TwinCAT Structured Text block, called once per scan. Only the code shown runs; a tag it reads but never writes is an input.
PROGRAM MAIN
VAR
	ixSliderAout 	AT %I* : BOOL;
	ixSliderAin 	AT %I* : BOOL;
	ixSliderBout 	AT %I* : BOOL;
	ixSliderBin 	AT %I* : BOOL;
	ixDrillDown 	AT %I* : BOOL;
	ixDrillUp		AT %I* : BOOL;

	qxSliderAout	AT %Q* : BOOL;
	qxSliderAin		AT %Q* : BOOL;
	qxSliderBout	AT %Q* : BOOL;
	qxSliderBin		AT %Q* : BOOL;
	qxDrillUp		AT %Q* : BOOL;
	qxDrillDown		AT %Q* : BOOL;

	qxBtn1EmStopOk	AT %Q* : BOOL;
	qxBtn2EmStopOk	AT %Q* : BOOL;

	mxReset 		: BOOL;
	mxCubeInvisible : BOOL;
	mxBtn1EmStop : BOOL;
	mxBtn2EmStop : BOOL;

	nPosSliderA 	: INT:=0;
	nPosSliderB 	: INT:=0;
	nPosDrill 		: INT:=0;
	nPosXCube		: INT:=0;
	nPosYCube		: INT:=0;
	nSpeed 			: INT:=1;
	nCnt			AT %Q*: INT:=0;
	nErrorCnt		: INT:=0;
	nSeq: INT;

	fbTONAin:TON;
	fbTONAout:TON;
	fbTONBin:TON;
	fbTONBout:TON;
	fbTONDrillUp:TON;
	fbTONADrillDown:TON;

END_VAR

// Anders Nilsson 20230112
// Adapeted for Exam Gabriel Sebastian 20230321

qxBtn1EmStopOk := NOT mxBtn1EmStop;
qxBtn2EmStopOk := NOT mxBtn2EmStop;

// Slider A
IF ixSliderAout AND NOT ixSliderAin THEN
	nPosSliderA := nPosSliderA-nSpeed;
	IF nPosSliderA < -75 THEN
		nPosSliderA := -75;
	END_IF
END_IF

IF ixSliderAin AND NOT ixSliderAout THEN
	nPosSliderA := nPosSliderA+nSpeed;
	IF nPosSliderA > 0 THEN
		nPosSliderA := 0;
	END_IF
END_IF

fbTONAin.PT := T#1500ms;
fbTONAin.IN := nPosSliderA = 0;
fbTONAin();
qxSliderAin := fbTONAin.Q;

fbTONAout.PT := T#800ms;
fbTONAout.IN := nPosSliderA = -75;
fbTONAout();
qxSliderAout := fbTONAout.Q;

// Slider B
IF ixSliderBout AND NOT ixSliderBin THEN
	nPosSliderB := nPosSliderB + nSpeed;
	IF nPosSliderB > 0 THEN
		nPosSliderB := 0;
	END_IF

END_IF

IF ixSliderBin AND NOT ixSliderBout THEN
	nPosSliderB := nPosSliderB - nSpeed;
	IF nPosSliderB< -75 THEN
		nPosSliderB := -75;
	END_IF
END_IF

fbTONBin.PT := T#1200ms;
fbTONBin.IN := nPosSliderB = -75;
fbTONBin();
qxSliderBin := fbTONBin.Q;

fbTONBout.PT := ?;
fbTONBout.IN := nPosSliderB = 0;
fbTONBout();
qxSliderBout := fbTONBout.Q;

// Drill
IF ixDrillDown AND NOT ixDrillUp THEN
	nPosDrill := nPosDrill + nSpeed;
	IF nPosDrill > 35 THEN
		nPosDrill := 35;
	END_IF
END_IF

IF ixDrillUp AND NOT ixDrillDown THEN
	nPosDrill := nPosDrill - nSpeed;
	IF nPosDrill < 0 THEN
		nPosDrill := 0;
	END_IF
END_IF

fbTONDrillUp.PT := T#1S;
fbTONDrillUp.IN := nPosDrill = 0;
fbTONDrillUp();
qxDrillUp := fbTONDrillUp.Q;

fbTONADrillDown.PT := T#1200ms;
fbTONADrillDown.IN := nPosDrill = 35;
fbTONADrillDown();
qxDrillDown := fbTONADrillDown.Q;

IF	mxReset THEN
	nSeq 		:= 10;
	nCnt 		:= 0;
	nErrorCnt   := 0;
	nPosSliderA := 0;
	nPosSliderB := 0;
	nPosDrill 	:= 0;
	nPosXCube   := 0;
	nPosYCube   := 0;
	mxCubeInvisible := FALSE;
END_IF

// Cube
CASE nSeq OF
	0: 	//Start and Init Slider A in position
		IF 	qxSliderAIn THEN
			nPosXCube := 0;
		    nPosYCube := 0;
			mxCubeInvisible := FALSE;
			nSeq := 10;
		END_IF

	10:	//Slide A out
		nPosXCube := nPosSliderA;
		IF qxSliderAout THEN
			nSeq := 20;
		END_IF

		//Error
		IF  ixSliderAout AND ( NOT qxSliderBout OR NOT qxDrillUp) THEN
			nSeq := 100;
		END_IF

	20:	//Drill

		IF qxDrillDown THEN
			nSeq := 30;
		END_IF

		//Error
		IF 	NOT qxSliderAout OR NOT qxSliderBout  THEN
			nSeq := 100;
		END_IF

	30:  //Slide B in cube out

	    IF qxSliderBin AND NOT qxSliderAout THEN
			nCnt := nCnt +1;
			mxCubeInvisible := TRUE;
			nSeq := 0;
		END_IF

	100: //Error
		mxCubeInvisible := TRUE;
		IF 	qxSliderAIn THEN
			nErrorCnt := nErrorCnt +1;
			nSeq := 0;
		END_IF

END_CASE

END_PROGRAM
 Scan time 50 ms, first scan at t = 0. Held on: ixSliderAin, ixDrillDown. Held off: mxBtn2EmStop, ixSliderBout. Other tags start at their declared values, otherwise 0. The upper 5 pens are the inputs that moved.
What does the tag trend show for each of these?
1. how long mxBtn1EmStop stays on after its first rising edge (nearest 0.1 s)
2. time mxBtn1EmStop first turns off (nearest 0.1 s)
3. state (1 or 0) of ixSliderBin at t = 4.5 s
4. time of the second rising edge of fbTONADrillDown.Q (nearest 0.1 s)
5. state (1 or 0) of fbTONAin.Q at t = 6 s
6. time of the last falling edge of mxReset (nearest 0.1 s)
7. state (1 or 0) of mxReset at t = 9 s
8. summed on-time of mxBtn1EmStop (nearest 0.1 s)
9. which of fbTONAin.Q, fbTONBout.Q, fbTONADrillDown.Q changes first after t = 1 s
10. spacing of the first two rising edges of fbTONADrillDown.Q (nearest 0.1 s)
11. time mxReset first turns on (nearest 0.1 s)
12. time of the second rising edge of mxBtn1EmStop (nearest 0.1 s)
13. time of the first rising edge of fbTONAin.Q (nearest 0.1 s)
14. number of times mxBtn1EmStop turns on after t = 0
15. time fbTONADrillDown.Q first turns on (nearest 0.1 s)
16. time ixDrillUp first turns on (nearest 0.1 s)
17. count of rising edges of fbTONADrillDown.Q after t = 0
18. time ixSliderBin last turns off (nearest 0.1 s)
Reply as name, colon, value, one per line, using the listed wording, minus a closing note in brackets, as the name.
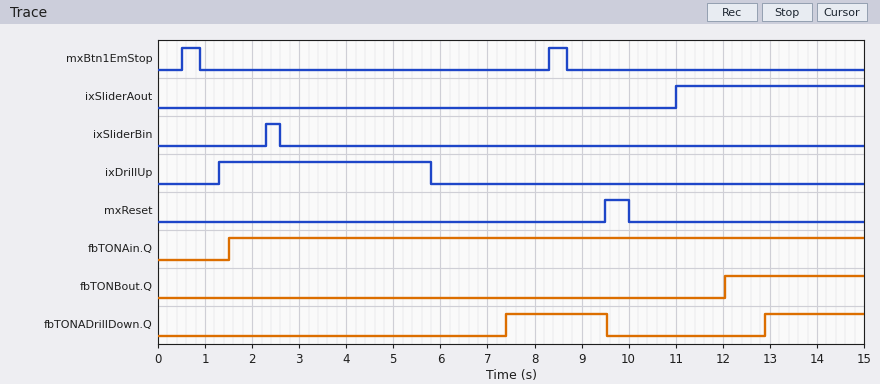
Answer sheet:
how long mxBtn1EmStop stays on after its first rising edge: 0.4 s
time mxBtn1EmStop first turns off: 0.9 s
state (1 or 0) of ixSliderBin at t = 4.5 s: 0
time of the second rising edge of fbTONADrillDown.Q: 12.9 s
state (1 or 0) of fbTONAin.Q at t = 6 s: 1
time of the last falling edge of mxReset: 10.0 s
state (1 or 0) of mxReset at t = 9 s: 0
summed on-time of mxBtn1EmStop: 0.8 s
which of fbTONAin.Q, fbTONBout.Q, fbTONADrillDown.Q changes first after t = 1 s: fbTONAin.Q
spacing of the first two rising edges of fbTONADrillDown.Q: 5.5 s
time mxReset first turns on: 9.5 s
time of the second rising edge of mxBtn1EmStop: 8.3 s
time of the first rising edge of fbTONAin.Q: 1.5 s
number of times mxBtn1EmStop turns on after t = 0: 2
time fbTONADrillDown.Q first turns on: 7.4 s
time ixDrillUp first turns on: 1.3 s
count of rising edges of fbTONADrillDown.Q after t = 0: 2
time ixSliderBin last turns off: 2.6 s
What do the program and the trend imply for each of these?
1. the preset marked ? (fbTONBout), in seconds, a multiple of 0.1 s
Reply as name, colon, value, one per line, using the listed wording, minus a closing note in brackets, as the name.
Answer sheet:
the preset marked ? (fbTONBout), in seconds, a multiple of 0.1 s: 2.5 s
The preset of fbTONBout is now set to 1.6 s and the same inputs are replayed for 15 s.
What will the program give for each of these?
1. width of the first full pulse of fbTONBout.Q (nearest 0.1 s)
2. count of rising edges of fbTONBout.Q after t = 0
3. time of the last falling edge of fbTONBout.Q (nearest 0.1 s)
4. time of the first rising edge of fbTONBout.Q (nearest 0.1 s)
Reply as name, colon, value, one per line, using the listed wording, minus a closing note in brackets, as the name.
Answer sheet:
width of the first full pulse of fbTONBout.Q: 0.7 s
count of rising edges of fbTONBout.Q after t = 0: 2
time of the last falling edge of fbTONBout.Q: 2.3 s
time of the first rising edge of fbTONBout.Q: 1.6 s
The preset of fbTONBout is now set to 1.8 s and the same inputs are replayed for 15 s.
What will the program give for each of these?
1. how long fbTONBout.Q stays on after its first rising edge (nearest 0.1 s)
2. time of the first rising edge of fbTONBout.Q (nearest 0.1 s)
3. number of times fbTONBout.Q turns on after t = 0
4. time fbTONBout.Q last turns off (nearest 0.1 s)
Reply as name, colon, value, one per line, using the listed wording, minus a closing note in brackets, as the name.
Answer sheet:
how long fbTONBout.Q stays on after its first rising edge: 0.5 s
time of the first rising edge of fbTONBout.Q: 1.8 s
number of times fbTONBout.Q turns on after t = 0: 2
time fbTONBout.Q last turns off: 2.3 s
